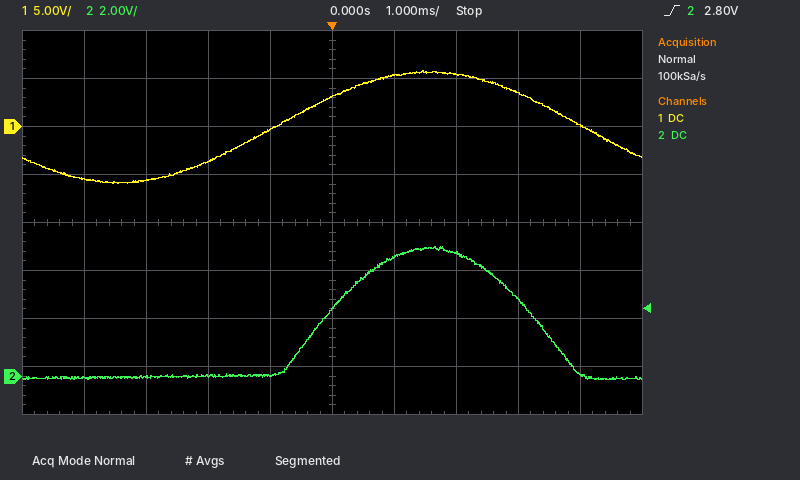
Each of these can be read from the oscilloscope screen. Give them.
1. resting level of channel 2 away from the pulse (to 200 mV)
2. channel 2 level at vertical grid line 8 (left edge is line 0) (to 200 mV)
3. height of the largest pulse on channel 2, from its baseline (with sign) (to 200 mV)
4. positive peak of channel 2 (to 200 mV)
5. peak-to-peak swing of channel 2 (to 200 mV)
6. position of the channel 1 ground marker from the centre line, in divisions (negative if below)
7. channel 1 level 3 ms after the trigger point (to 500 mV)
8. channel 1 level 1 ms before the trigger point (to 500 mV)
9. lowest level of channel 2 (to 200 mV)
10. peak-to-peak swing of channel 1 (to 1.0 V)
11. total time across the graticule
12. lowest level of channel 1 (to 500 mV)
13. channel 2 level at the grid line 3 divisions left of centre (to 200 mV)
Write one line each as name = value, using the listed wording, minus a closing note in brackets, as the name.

resting level of channel 2 away from the pulse = 0.0 V
channel 2 level at vertical grid line 8 (left edge is line 0) = 3.2 V
height of the largest pulse on channel 2, from its baseline (with sign) = +5.4 V
positive peak of channel 2 = 5.4 V
peak-to-peak swing of channel 2 = 5.6 V
position of the channel 1 ground marker from the centre line, in divisions = +2.0 div
channel 1 level 3 ms after the trigger point = 3.5 V
channel 1 level 1 ms before the trigger point = -500 mV
lowest level of channel 2 = -200 mV
peak-to-peak swing of channel 1 = 12.0 V
total time across the graticule = 10 ms
lowest level of channel 1 = -6.0 V
channel 2 level at the grid line 3 divisions left of centre = 0.0 V
